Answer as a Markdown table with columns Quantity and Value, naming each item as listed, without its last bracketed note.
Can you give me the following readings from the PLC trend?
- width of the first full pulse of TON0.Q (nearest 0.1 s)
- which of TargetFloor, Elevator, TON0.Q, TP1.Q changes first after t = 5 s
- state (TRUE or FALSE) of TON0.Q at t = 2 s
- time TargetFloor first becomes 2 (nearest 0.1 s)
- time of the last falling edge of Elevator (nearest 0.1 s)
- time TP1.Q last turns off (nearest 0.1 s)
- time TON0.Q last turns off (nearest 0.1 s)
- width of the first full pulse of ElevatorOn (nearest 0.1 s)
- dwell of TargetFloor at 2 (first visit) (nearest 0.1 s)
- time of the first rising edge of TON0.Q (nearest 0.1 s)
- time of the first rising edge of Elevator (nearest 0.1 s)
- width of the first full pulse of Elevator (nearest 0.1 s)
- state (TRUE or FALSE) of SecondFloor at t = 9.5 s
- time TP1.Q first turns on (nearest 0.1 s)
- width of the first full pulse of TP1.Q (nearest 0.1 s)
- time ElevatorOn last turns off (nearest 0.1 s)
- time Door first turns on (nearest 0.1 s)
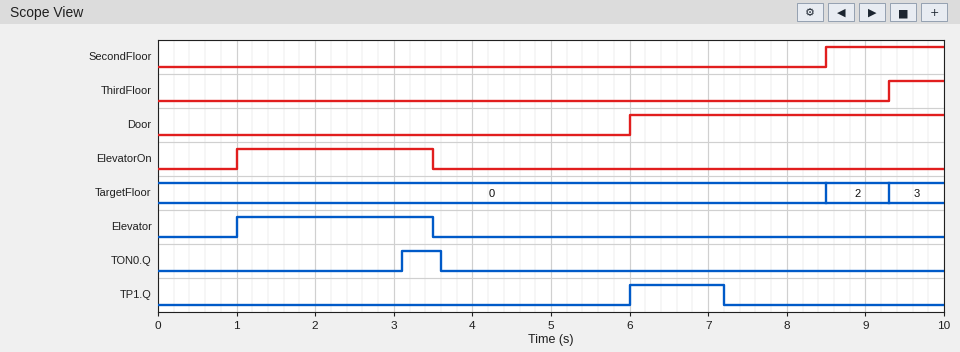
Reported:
| Quantity | Value |
|---|---|
| width of the first full pulse of TON0.Q | 0.5 s |
| which of TargetFloor, Elevator, TON0.Q, TP1.Q changes first after t = 5 s | TP1.Q |
| state (TRUE or FALSE) of TON0.Q at t = 2 s | FALSE |
| time TargetFloor first becomes 2 | 8.5 s |
| time of the last falling edge of Elevator | 3.5 s |
| time TP1.Q last turns off | 7.2 s |
| time TON0.Q last turns off | 3.6 s |
| width of the first full pulse of ElevatorOn | 2.5 s |
| dwell of TargetFloor at 2 (first visit) | 0.8 s |
| time of the first rising edge of TON0.Q | 3.1 s |
| time of the first rising edge of Elevator | 1.0 s |
| width of the first full pulse of Elevator | 2.5 s |
| state (TRUE or FALSE) of SecondFloor at t = 9.5 s | TRUE |
| time TP1.Q first turns on | 6.0 s |
| width of the first full pulse of TP1.Q | 1.2 s |
| time ElevatorOn last turns off | 3.5 s |
| time Door first turns on | 6.0 s |
